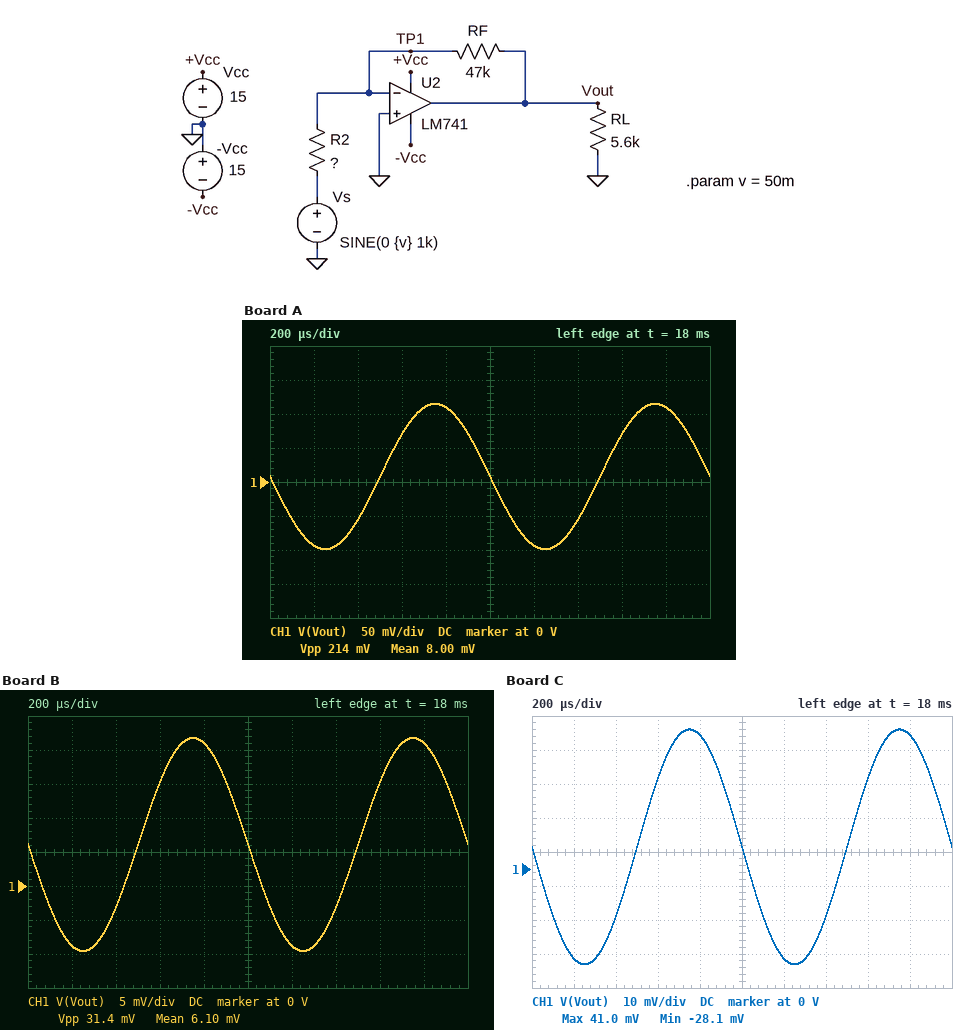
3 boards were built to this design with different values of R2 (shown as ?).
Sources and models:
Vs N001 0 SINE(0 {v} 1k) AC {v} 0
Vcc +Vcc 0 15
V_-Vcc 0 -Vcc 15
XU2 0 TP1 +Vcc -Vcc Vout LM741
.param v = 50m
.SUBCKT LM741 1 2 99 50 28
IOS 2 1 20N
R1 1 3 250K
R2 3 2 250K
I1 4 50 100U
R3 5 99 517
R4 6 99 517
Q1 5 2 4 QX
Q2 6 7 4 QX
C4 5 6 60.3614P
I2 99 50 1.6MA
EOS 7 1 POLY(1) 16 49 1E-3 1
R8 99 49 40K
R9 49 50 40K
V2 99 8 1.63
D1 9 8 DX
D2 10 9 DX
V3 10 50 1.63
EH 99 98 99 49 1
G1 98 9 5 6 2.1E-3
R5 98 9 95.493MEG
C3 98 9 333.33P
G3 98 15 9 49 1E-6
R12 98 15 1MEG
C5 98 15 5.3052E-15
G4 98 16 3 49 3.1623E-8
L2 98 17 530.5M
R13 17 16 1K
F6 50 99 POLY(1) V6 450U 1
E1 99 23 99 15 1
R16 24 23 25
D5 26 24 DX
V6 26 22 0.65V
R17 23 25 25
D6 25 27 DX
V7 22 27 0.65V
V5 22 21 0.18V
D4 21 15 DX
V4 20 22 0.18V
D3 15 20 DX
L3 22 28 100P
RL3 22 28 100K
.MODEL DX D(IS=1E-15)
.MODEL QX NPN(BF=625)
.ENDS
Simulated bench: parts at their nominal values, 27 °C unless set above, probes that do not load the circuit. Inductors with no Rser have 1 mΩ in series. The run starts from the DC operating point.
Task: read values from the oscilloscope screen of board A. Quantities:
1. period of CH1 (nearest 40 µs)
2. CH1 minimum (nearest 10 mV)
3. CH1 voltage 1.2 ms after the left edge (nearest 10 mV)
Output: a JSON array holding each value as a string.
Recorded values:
["1.00 ms", "-100 mV", "-90 mV"]
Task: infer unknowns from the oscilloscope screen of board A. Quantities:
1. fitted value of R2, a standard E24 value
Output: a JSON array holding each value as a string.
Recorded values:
["22 kΩ"]
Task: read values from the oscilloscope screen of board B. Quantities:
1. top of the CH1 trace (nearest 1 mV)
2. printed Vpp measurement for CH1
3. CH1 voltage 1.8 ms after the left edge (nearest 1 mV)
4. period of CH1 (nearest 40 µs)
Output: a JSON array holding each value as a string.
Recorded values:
["22 mV", "31.4 mV", "21 mV", "1.00 ms"]
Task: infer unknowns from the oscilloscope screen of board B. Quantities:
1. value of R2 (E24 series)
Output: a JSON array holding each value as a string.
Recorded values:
["150 kΩ"]
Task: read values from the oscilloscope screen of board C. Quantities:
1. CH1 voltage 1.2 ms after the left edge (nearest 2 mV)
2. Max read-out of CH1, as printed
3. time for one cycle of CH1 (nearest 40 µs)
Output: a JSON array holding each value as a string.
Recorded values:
["-26 mV", "41.0 mV", "1.00 ms"]
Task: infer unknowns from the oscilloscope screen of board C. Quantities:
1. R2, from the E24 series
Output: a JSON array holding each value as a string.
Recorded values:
["68 kΩ"]
